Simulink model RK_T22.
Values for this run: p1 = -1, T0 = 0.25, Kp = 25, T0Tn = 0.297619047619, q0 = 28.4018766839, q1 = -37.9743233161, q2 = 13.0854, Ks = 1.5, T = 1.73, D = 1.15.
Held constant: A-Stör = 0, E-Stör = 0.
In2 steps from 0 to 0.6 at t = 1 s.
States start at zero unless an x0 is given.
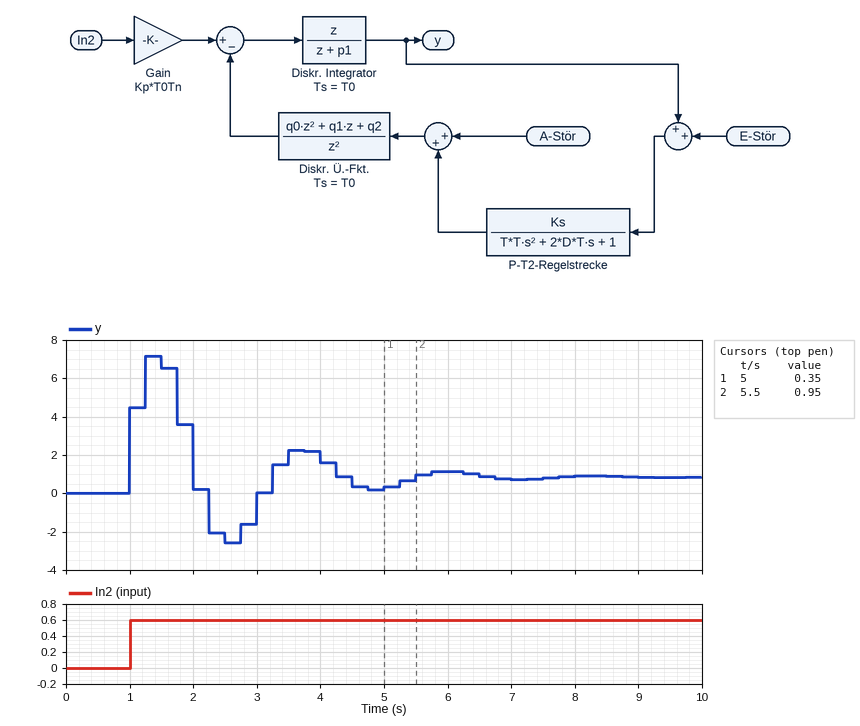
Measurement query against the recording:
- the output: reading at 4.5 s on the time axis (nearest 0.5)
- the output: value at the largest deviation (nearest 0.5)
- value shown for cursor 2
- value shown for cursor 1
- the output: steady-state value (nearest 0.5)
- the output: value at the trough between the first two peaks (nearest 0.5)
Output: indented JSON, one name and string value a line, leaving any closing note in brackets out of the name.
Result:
{
  "the output: reading at 4.5 s on the time axis": "0.5",
  "the output: value at the largest deviation": "7.0",
  "value shown for cursor 2": "0.95",
  "value shown for cursor 1": "0.35",
  "the output: steady-state value": "1.0",
  "the output: value at the trough between the first two peaks": "-2.5"
}
